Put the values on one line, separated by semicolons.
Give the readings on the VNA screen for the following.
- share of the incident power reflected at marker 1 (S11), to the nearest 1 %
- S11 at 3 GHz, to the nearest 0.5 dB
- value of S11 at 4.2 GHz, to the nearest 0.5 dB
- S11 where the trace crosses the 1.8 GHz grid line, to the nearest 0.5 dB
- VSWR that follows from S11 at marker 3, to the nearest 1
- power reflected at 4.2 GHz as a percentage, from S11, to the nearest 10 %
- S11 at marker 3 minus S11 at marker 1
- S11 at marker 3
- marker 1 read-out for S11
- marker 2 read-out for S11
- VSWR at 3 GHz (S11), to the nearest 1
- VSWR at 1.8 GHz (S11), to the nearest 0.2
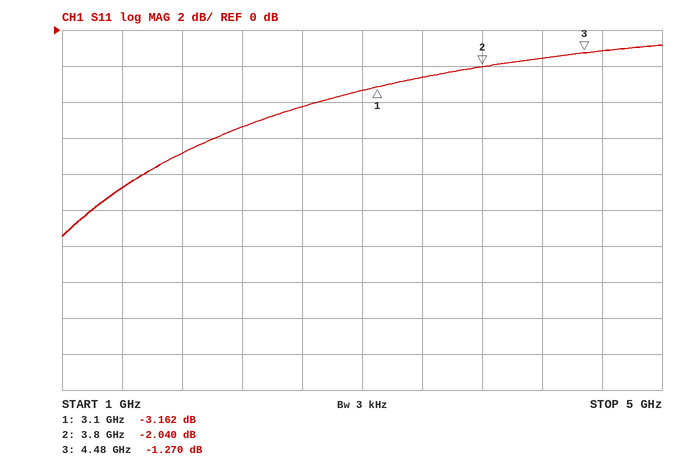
48 %; -3.5 dB; -1.5 dB; -7.0 dB; 14; 70 %; 1.892 dB; -1.270 dB; -3.162 dB; -2.040 dB; 5; 2.6
